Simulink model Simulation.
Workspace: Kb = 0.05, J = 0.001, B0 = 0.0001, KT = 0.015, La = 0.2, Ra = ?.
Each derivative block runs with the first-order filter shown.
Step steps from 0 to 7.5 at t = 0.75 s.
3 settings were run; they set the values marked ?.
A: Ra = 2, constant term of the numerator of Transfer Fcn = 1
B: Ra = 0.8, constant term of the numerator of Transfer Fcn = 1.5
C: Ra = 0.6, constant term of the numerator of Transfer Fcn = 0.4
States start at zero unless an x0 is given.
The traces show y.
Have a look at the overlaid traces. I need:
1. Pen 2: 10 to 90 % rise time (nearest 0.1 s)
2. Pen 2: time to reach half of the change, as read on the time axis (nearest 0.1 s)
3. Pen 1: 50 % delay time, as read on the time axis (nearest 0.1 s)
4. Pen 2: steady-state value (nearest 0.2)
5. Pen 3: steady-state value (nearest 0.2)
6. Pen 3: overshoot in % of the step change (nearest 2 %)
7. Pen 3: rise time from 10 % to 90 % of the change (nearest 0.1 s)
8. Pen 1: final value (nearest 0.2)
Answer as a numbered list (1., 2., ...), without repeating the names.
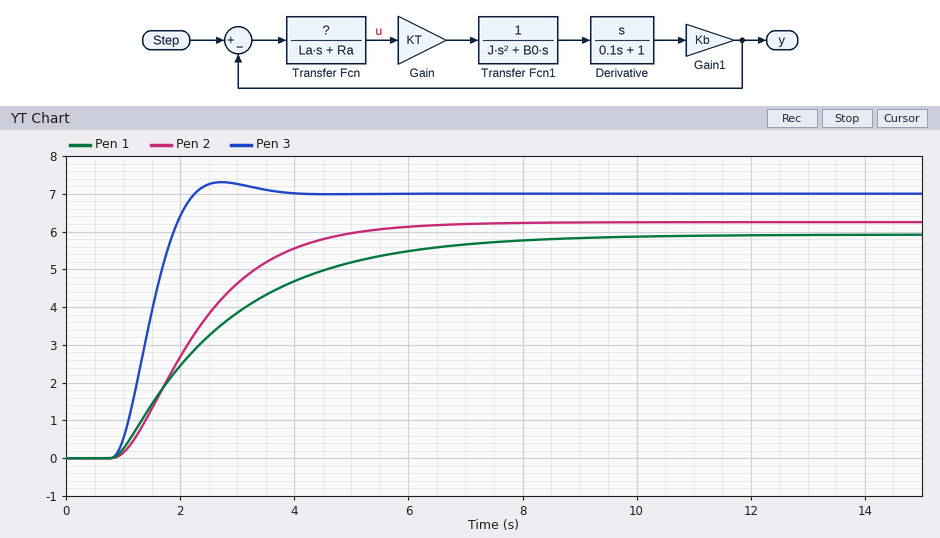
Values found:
1. 2.9 s
2. 2.2 s
3. 2.3 s
4. 6.2
5. 7.0
6. 4 %
7. 0.9 s
8. 6.0
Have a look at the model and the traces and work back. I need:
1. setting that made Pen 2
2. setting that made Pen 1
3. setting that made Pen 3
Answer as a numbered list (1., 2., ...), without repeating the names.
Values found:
1. C
2. A
3. B
